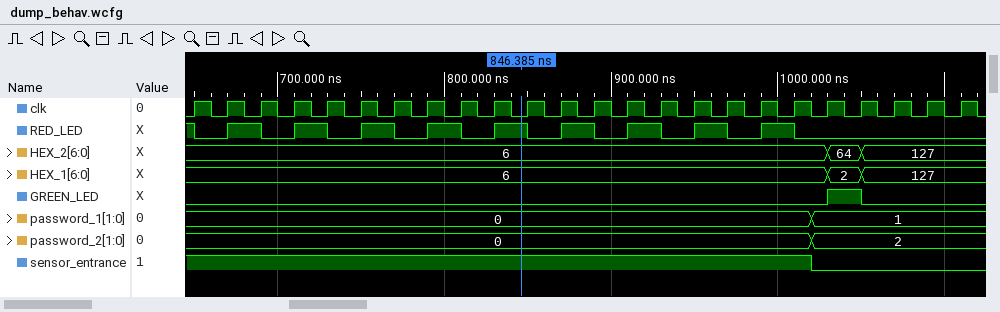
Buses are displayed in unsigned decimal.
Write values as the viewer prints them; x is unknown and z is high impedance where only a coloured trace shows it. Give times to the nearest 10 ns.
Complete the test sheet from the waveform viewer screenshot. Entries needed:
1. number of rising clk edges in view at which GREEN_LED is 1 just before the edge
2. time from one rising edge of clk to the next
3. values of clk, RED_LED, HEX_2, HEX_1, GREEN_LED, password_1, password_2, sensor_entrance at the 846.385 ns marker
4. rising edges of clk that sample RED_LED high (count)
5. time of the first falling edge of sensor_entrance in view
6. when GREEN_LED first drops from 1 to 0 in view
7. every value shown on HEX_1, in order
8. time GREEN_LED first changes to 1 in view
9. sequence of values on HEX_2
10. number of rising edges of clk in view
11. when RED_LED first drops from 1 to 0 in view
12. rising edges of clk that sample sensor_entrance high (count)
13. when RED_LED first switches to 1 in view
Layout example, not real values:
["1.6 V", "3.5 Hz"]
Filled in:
["1", "20 ns", "clk=0, RED_LED=1, HEX_2=6, HEX_1=6, GREEN_LED=0, password_1=0, password_2=0, sensor_entrance=1", "10", "1020 ns", "1050 ns", "6, 2, 127", "1030 ns", "6, 64, 127", "24", "650 ns", "19", "670 ns"]
